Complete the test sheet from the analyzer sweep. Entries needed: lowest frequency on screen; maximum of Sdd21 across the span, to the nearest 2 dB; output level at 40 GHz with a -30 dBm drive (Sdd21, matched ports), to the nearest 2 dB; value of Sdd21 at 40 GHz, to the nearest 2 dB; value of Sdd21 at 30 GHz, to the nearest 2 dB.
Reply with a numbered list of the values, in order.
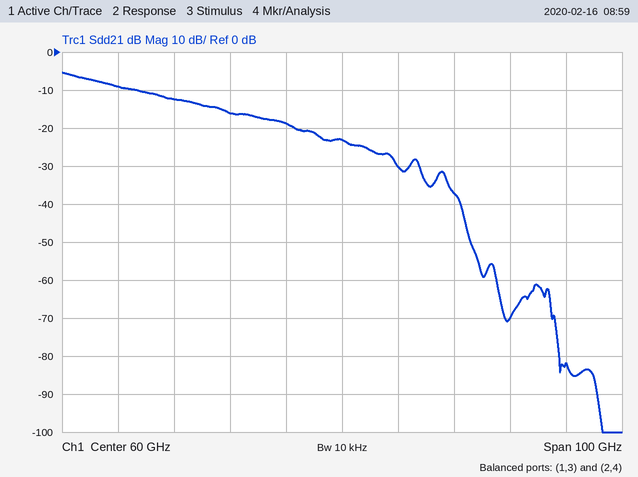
1. 10 GHz
2. -6 dB
3. -46 dBm
4. -16 dB
5. -12 dB
